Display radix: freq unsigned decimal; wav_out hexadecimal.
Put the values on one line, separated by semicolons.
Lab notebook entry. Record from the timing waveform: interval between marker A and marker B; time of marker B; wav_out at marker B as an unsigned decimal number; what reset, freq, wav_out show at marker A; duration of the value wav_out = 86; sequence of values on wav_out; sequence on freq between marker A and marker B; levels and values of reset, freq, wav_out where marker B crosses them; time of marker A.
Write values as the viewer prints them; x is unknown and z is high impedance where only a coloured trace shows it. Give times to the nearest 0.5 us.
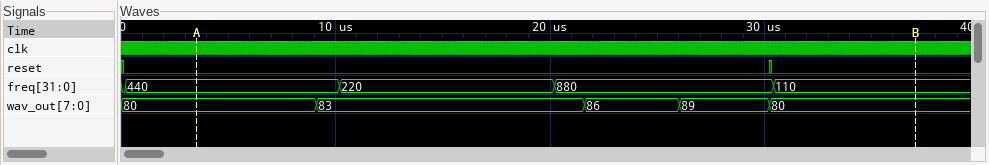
33.5 us; 37 us; 128; reset=0, freq=440, wav_out=80; 4.5 us; 80, 83, 86, 89, 80; 440, 220, 880, 110; reset=0, freq=110, wav_out=80; 3.5 us
